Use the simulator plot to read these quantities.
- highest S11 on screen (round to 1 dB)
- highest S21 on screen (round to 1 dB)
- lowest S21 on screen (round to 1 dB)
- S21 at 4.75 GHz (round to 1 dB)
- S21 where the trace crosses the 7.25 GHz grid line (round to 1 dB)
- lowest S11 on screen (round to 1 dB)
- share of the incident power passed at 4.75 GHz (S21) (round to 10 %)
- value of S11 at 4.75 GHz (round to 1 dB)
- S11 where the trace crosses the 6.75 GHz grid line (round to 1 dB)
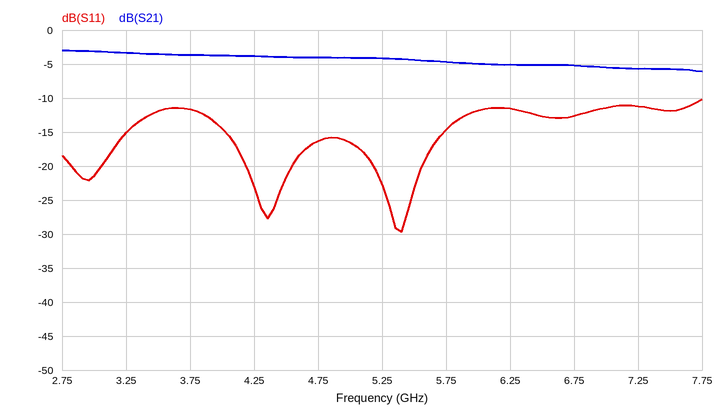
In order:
-10 dB
-3 dB
-6 dB
-4 dB
-6 dB
-30 dB
40 %
-16 dB
-13 dB
